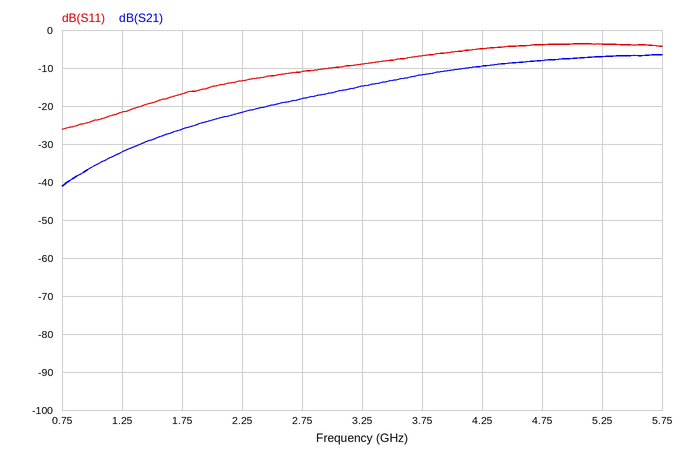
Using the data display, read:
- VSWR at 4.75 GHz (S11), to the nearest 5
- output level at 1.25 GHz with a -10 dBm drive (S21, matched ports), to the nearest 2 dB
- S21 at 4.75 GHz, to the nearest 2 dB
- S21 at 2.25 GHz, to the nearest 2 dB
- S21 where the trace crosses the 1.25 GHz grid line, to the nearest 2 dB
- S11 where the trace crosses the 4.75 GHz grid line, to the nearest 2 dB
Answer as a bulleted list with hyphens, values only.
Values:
- 5
- -42 dBm
- -8 dB
- -22 dB
- -32 dB
- -4 dB
